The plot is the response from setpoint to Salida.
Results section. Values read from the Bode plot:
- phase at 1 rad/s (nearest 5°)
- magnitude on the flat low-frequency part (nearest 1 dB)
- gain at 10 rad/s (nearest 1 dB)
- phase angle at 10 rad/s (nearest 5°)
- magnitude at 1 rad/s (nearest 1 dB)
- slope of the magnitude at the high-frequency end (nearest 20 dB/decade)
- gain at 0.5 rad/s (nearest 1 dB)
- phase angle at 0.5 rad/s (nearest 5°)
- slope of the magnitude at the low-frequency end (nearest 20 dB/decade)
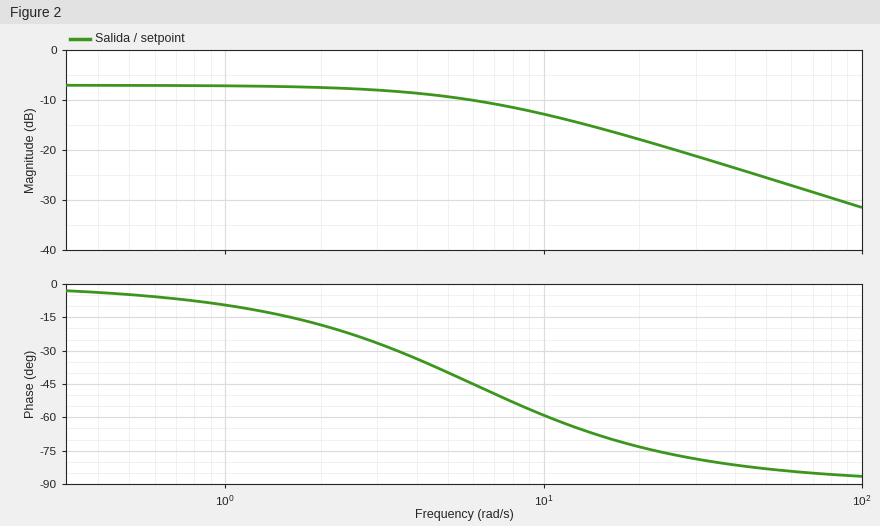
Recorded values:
-10°
-7 dB
-13 dB
-60°
-7 dB
-20 dB/decade
-7 dB
-5°
0 dB/decade
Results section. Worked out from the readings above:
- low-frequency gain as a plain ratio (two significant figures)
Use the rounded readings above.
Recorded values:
0.45
